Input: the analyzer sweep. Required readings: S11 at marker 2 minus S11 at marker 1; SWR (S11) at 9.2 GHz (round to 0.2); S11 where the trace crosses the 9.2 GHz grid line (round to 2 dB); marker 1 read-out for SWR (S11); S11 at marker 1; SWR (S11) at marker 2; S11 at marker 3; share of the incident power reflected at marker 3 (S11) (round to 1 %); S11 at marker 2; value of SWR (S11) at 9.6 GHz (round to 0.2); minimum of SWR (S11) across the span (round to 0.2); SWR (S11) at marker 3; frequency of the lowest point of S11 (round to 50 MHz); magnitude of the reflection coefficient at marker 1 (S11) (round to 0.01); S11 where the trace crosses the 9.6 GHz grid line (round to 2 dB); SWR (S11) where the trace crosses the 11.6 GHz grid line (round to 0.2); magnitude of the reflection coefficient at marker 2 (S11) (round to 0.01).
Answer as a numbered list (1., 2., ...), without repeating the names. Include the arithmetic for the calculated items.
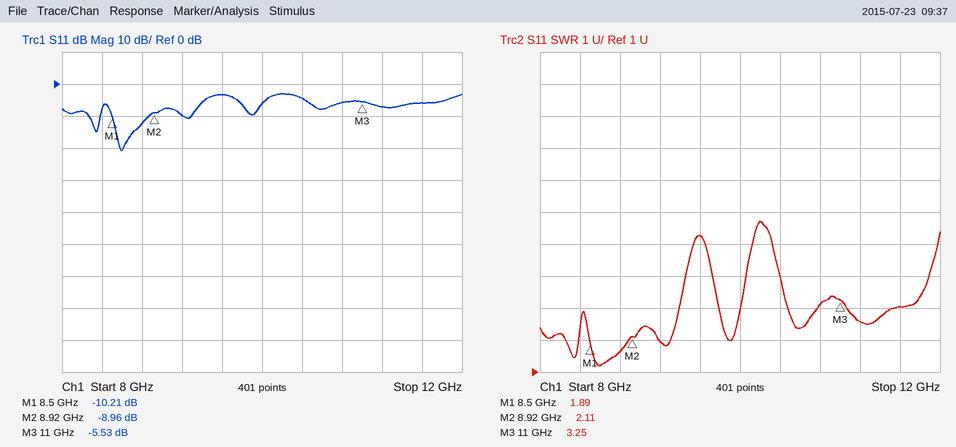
1. -8.96 − (-10.21) = 1.25 dB
2. 2.0
3. -10 dB
4. 1.89
5. -10.21 dB
6. 2.11
7. -5.53 dB
8. 10^(-5.53/10) ≈ 28 %
9. -8.96 dB
10. 5.2
11. 1.2
12. 3.25
13. 8.60 GHz
14. 10^(-10.21/20) ≈ 0.31
15. -4 dB
16. 3.0
17. 10^(-8.96/20) ≈ 0.36
